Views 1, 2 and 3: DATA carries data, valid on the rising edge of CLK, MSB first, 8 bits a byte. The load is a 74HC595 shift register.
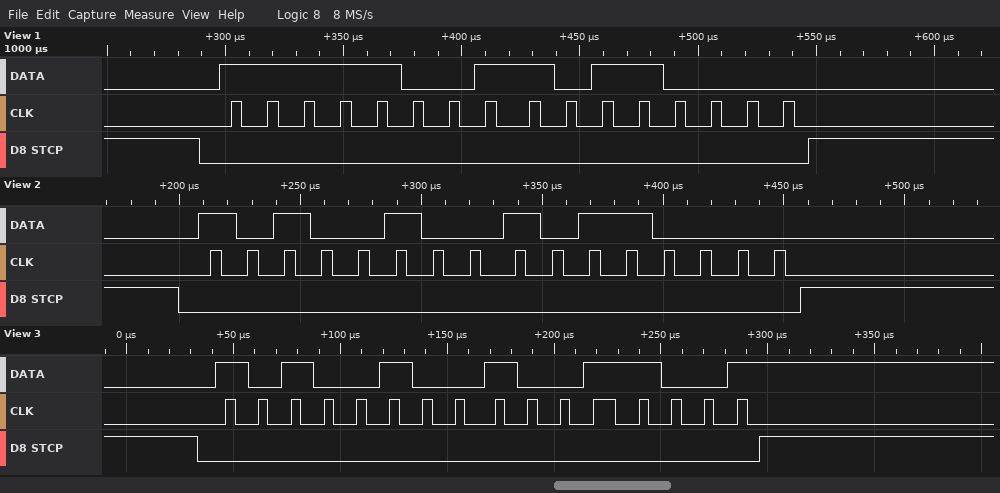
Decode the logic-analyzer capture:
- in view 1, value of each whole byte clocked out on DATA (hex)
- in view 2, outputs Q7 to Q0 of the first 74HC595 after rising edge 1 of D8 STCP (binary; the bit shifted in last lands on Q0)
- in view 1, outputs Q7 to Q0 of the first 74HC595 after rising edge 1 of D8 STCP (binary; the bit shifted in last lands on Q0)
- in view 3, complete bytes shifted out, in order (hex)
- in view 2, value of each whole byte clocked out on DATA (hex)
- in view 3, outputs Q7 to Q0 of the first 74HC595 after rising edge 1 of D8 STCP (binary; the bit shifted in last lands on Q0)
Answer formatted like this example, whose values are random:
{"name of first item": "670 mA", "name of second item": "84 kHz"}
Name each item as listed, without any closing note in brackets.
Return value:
{"in view 1, value of each whole byte clocked out on DATA": "F9 B0", "in view 2, outputs Q7 to Q0 of the first 74HC595 after rising edge 1 of D8 STCP": "10110000", "in view 1, outputs Q7 to Q0 of the first 74HC595 after rising edge 1 of D8 STCP": "10110000", "in view 3, complete bytes shifted out, in order": "A4 99", "in view 2, value of each whole byte clocked out on DATA": "0xA4 0xB0", "in view 3, outputs Q7 to Q0 of the first 74HC595 after rising edge 1 of D8 STCP": "10011001"}
